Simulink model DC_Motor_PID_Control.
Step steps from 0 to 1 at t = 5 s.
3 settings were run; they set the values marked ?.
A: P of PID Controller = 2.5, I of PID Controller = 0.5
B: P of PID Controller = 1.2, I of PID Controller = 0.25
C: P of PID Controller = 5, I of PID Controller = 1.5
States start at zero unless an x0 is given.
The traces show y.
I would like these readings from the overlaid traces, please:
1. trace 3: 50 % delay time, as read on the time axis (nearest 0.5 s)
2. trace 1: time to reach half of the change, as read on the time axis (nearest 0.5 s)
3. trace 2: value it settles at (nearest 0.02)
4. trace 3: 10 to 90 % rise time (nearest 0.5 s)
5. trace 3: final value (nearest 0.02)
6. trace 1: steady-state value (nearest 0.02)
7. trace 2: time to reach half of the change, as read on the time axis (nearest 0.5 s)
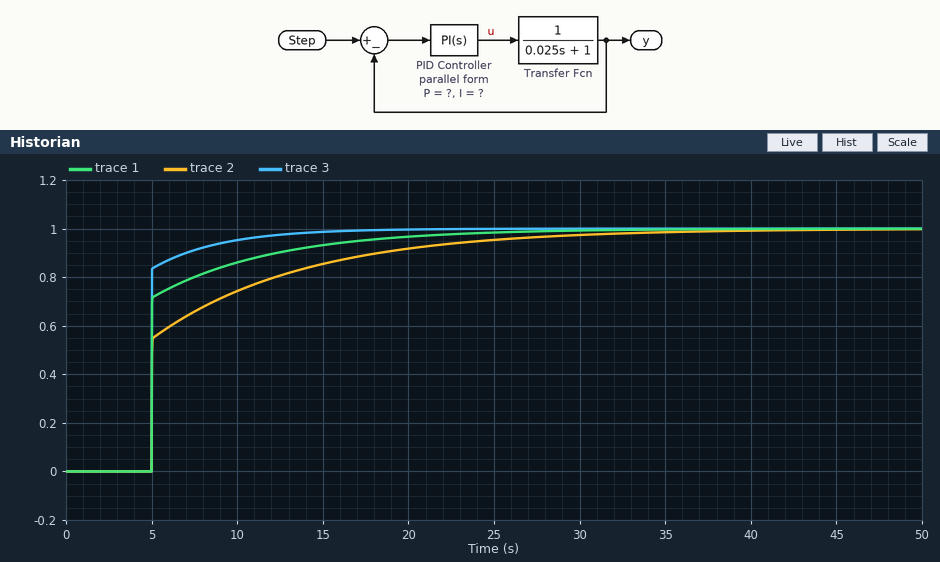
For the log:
5.0 s
5.0 s
1.00
2.0 s
1.00
1.00
5.0 s
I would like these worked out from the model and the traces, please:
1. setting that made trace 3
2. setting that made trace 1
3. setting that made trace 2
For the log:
C
A
B
